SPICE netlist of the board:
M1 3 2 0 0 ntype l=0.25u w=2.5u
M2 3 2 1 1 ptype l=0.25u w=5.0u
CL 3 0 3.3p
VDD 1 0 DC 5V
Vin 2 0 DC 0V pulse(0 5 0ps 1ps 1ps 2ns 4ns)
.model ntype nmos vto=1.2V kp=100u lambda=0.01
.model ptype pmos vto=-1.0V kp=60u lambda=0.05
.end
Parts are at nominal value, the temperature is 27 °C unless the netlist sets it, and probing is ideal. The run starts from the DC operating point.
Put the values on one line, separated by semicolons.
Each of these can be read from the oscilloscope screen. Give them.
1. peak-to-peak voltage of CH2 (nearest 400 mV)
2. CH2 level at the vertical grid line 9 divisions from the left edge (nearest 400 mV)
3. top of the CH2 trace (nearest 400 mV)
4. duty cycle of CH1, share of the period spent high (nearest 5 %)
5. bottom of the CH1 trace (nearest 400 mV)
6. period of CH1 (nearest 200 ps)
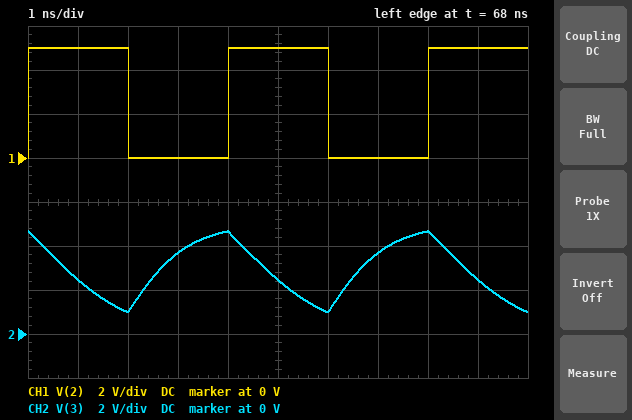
3.6 V; 2.4 V; 4.8 V; 50 %; 0 V; 4.0 ns
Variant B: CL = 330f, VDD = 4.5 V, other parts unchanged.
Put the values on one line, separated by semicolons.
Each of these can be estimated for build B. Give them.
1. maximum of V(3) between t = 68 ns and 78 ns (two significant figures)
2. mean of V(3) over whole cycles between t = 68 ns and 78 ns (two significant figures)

4.5 V; 2.3 V
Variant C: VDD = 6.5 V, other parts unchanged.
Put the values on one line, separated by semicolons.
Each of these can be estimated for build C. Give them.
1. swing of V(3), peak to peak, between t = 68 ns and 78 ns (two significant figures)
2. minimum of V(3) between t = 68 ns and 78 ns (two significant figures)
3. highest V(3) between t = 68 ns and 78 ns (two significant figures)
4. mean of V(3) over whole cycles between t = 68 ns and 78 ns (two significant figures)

4.3 V; 2.1 V; 6.4 V; 4.7 V
